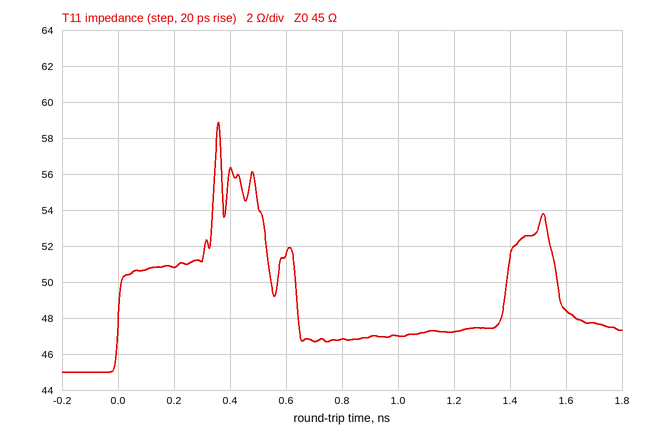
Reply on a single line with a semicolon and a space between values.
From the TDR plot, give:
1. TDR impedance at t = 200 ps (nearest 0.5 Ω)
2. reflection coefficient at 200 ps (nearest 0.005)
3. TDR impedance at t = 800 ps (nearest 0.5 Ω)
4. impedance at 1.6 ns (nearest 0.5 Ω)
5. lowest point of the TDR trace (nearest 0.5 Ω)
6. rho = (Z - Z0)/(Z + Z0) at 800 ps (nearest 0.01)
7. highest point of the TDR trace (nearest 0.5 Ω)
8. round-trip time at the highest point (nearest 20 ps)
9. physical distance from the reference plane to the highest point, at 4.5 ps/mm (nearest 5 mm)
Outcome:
51.0 Ω; +0.060; 47.0 Ω; 48.5 Ω; 45.0 Ω; +0.02; 59.0 Ω; 360 ps; 40 mm
